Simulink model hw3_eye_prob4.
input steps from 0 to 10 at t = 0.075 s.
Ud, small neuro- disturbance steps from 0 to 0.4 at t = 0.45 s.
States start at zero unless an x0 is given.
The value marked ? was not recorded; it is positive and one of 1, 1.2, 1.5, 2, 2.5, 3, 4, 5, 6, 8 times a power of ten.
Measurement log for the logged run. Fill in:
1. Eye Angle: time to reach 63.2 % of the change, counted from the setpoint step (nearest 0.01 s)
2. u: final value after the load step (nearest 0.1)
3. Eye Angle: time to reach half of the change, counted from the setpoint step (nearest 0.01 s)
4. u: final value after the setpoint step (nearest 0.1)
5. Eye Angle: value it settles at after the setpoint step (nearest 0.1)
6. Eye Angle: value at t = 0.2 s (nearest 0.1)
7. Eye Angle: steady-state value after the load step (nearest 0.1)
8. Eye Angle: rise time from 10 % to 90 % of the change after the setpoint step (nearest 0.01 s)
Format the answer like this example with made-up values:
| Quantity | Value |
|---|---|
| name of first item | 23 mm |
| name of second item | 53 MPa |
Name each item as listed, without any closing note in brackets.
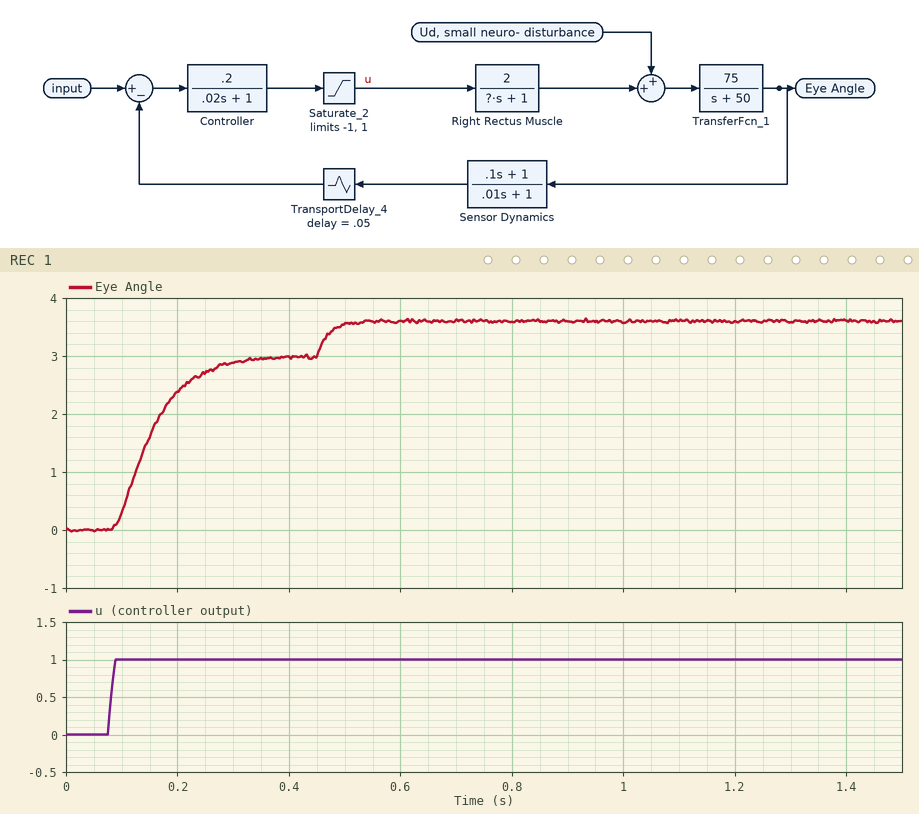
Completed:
| Quantity | Value |
|---|---|
| Eye Angle: time to reach 63.2 % of the change, counted from the setpoint step | 0.09 s |
| u: final value after the load step | 1.0 |
| Eye Angle: time to reach half of the change, counted from the setpoint step | 0.07 s |
| u: final value after the setpoint step | 1.0 |
| Eye Angle: value it settles at after the setpoint step | 3.0 |
| Eye Angle: value at t = 0.2 s | 2.4 |
| Eye Angle: steady-state value after the load step | 3.6 |
| Eye Angle: rise time from 10 % to 90 % of the change after the setpoint step | 0.14 s |
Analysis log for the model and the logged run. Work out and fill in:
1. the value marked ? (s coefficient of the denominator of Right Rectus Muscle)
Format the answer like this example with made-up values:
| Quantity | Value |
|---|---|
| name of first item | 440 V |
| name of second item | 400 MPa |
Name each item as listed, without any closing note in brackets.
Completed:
| Quantity | Value |
|---|---|
| the value marked ? | 0.06 |
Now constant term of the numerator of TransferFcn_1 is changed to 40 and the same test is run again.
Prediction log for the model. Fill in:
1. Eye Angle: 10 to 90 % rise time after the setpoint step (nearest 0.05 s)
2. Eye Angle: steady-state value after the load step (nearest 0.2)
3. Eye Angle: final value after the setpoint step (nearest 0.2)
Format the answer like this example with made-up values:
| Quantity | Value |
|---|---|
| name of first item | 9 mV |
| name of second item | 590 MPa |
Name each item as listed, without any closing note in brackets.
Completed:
| Quantity | Value |
|---|---|
| Eye Angle: 10 to 90 % rise time after the setpoint step | 0.15 s |
| Eye Angle: steady-state value after the load step | 2.0 |
| Eye Angle: final value after the setpoint step | 1.6 |
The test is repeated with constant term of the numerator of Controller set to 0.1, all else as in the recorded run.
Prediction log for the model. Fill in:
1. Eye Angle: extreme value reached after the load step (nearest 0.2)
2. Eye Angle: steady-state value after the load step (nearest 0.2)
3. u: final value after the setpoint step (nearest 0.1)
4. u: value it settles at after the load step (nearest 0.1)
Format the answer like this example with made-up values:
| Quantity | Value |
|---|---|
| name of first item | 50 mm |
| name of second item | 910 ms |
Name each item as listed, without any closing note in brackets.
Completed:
| Quantity | Value |
|---|---|
| Eye Angle: extreme value reached after the load step | 2.8 |
| Eye Angle: steady-state value after the load step | 2.8 |
| u: final value after the setpoint step | 0.8 |
| u: value it settles at after the load step | 0.7 |
